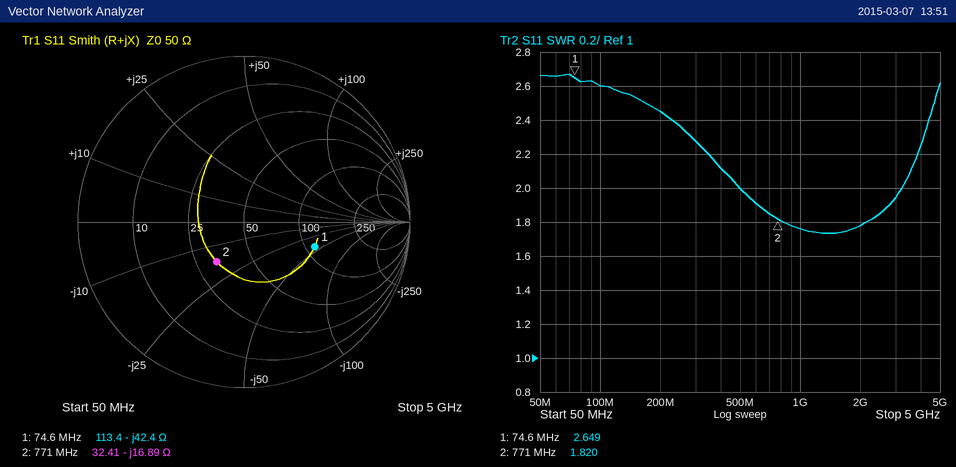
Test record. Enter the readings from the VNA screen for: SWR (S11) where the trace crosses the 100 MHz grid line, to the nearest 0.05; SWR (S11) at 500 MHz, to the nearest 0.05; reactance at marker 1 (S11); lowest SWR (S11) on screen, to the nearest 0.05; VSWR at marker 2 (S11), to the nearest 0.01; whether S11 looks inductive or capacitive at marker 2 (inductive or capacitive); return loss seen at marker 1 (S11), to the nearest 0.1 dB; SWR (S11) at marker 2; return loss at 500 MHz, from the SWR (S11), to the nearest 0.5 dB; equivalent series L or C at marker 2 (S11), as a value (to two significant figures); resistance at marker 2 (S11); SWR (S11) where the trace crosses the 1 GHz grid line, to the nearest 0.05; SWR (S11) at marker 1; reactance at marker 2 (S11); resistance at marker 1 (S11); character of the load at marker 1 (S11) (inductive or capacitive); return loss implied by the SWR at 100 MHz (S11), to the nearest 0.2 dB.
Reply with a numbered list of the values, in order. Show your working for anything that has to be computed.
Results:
1. 2.60
2. 2.00
3. -42.4 Ω
4. 1.75
5. 1.82
6. capacitive
7. 6.9 dB
8. 1.820
9. −20 log10((2 − 1)/(2 + 1)) ≈ 9.5 dB
10. C = 1/(2π × 771 MHz × 16.89 Ω) ≈ 12 pF
11. 32.41 Ω
12. 1.75
13. 2.649
14. -16.89 Ω
15. 113.4 Ω
16. capacitive
17. −20 log10((2.6 − 1)/(2.6 + 1)) ≈ 7.0 dB
